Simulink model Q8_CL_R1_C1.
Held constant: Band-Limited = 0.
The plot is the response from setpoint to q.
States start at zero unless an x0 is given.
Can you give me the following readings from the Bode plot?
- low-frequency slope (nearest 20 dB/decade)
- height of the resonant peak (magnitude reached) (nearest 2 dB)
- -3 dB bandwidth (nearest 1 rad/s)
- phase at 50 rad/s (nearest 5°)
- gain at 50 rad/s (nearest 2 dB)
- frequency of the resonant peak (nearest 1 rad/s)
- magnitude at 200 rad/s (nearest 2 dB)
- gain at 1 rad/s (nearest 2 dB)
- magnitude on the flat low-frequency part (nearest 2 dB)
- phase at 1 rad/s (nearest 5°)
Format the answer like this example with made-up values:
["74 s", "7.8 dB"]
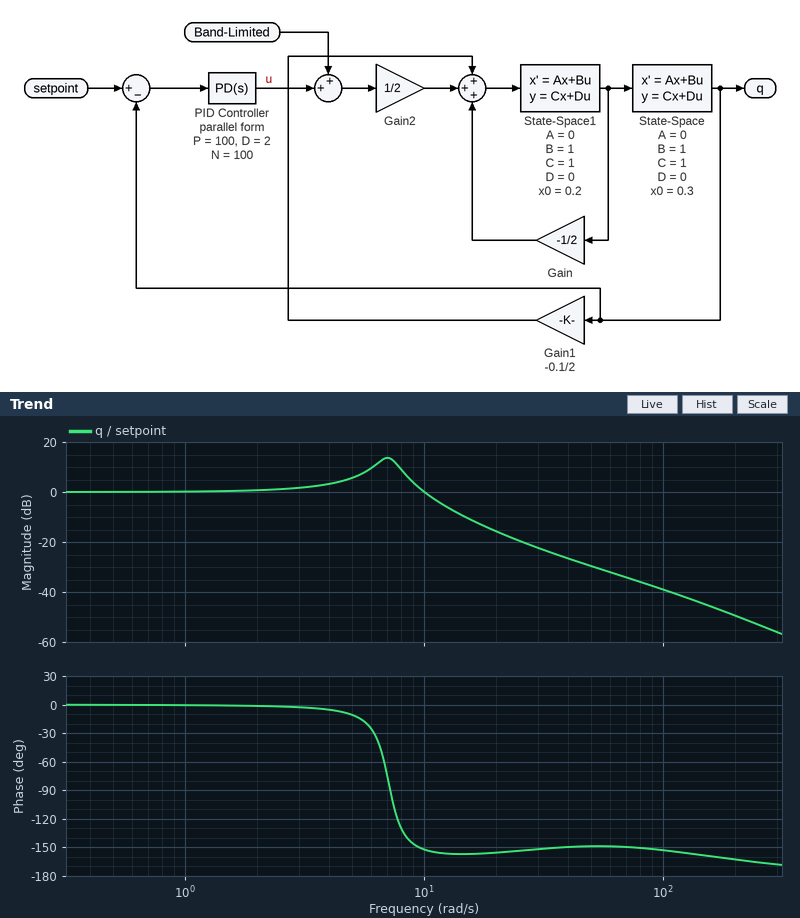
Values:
["0 dB/decade", "14 dB", "11 rad/s", "-150°", "-30 dB", "7 rad/s", "-50 dB", "0 dB", "0 dB", "0°"]
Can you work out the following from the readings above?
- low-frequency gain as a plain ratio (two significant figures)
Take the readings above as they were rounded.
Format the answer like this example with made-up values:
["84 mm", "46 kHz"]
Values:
["1.0"]
